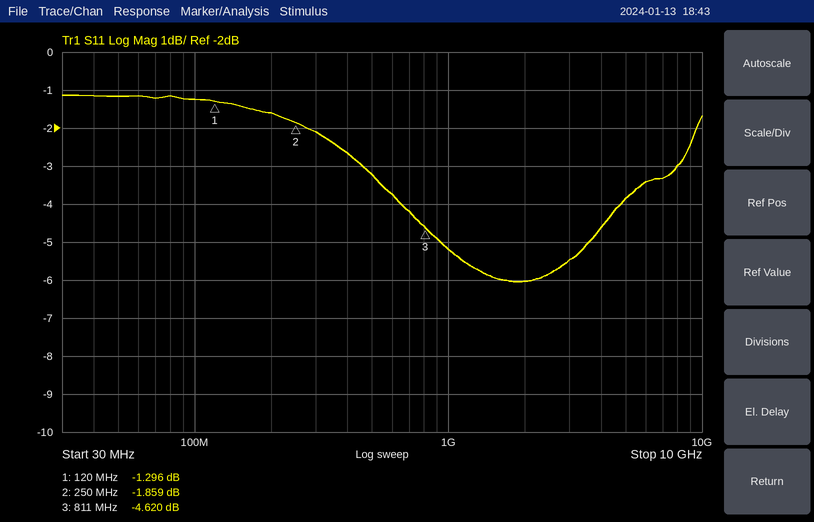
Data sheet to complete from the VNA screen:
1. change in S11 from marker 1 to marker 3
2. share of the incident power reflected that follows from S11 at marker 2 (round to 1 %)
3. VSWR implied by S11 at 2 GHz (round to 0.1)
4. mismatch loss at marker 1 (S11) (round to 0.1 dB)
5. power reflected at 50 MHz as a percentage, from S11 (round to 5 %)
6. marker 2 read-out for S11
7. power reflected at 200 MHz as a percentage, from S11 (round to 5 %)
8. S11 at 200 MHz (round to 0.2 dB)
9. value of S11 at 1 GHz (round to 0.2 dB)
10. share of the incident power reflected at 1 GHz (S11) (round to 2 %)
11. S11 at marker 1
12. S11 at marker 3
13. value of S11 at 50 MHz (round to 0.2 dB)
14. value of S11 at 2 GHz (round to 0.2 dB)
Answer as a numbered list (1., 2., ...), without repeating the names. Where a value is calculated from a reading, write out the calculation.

1. -4.62 − (-1.296) = -3.324 dB
2. 10^(-1.859/10) ≈ 65 %
3. |Γ| = 10^(-6/20) = 0.5012; VSWR = (1 + 0.5012)/(1 − 0.5012) ≈ 3.0
4. −10 log10(1 − 10^(-1.296/10)) ≈ 5.9 dB
5. 10^(-1.2/10) ≈ 75.9 %, so 75 % to the nearest 5 %
6. -1.859 dB
7. 10^(-1.6/10) ≈ 69.2 %, so 70 % to the nearest 5 %
8. -1.6 dB
9. -5.2 dB
10. 10^(-5.2/10) ≈ 30 %
11. -1.296 dB
12. -4.620 dB
13. -1.2 dB
14. -6.0 dB
